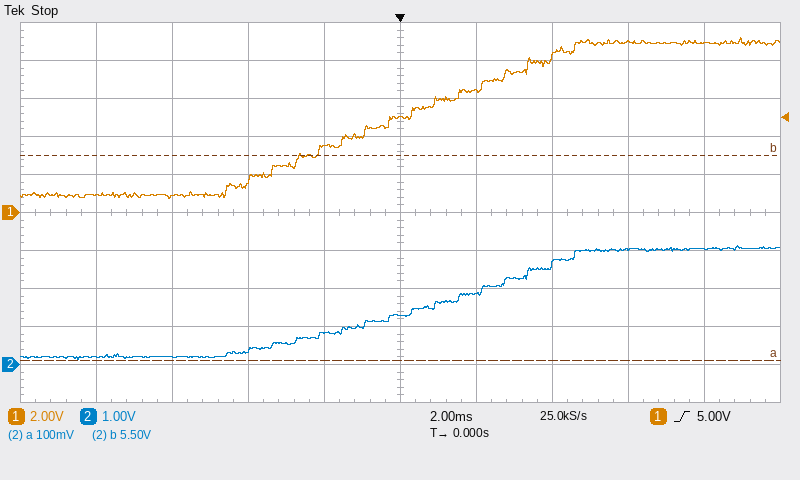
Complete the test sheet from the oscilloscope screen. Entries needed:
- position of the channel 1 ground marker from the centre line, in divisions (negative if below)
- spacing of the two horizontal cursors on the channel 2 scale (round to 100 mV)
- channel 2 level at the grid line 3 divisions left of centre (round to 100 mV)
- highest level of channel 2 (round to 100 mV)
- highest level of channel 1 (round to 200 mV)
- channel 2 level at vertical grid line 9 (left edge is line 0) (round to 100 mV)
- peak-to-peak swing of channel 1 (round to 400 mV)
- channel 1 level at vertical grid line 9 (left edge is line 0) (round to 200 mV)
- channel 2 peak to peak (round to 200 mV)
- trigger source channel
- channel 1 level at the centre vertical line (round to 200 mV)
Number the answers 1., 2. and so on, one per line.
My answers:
1. 0.0 div
2. 5.4 V
3. 200 mV
4. 3.1 V
5. 9.2 V
6. 3.0 V
7. 8.4 V
8. 9.0 V
9. 3.0 V
10. channel 1
11. 5.0 V
